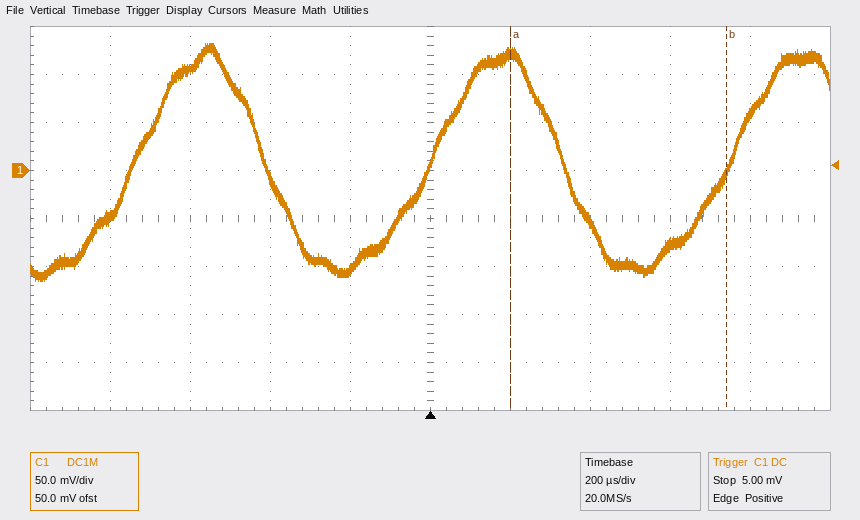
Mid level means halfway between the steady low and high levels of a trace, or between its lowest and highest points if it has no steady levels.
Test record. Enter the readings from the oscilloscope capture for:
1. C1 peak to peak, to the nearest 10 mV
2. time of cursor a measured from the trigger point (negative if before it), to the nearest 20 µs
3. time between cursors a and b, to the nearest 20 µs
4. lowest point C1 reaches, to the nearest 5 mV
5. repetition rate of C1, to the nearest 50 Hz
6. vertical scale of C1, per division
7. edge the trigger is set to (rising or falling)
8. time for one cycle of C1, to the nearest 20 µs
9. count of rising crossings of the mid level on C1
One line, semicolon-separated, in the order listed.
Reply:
250 mV; +200 µs; 540 µs; -115 mV; 1.35 kHz; 50 mV; rising; 740 µs; 3
